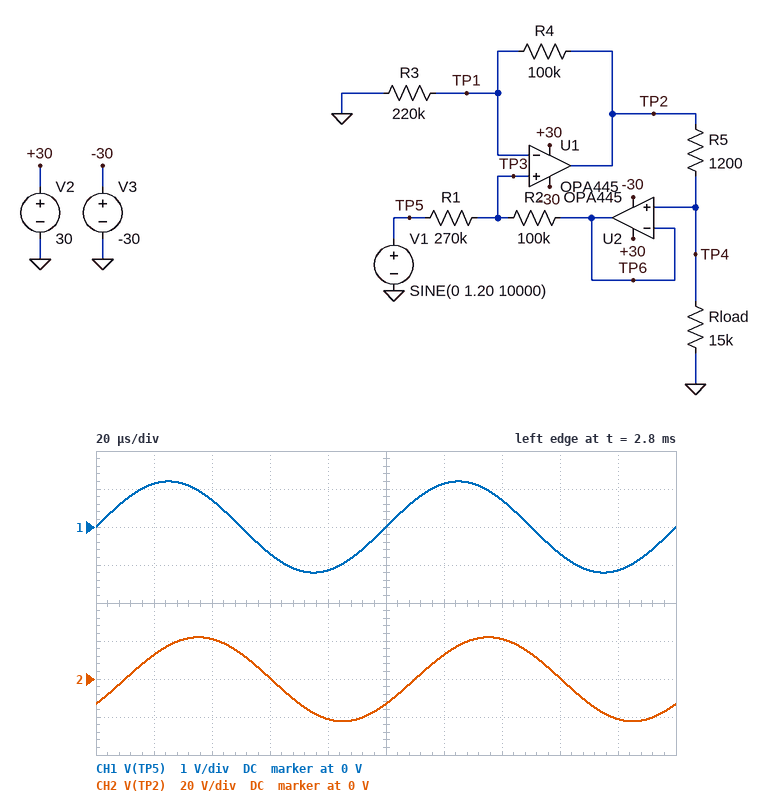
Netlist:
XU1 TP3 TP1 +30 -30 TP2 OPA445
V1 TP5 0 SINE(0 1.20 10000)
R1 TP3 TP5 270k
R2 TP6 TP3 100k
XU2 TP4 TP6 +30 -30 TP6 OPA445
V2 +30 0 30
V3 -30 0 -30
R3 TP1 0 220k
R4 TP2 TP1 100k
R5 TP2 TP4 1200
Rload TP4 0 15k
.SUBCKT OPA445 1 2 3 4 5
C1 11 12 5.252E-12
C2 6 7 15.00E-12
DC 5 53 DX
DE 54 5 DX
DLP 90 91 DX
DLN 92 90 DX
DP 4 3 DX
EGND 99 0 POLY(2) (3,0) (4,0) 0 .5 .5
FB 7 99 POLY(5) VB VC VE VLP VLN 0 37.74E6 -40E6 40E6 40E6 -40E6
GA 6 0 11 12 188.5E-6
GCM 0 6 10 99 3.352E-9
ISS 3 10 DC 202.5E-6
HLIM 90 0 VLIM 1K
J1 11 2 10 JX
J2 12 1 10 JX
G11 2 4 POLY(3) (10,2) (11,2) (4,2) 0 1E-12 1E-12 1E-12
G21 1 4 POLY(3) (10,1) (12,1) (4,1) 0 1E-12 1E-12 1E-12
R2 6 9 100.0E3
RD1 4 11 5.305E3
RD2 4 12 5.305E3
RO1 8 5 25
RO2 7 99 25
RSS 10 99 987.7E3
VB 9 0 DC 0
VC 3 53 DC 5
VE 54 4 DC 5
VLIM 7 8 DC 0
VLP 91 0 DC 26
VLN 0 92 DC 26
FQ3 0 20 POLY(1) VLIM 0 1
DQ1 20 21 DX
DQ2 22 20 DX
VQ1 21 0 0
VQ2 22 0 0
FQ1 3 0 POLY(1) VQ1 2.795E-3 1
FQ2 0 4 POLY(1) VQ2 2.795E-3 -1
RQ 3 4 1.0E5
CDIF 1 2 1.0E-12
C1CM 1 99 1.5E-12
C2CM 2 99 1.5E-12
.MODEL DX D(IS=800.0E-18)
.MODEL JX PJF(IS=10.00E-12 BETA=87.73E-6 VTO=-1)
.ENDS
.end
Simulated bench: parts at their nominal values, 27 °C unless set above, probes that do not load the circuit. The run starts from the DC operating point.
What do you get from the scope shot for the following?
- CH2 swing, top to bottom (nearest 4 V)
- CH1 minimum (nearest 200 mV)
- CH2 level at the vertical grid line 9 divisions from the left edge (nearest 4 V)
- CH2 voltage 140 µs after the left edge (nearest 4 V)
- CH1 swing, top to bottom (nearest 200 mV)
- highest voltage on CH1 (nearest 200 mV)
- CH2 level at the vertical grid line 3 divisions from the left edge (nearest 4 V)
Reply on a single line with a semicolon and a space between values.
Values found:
44 V; -1.2 V; -20 V; 20 V; 2.4 V; 1.2 V; 0 V
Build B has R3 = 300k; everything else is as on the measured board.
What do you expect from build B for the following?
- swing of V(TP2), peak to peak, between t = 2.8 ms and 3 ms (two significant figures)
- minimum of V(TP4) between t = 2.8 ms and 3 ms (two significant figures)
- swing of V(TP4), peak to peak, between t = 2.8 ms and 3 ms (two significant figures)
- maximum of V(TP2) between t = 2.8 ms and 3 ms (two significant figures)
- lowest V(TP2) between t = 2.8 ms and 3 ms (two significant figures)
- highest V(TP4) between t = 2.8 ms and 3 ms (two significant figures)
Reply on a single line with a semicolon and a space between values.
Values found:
8.7 V; -4.0 V; 8.0 V; 4.3 V; -4.3 V; 4.0 V
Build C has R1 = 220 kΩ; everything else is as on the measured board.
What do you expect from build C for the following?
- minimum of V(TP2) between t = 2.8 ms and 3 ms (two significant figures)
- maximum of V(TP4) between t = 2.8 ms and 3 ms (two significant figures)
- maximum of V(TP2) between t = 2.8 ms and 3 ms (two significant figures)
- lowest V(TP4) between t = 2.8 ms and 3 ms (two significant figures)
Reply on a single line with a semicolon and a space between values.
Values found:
-7.3 V; 6.7 V; 7.3 V; -6.7 V
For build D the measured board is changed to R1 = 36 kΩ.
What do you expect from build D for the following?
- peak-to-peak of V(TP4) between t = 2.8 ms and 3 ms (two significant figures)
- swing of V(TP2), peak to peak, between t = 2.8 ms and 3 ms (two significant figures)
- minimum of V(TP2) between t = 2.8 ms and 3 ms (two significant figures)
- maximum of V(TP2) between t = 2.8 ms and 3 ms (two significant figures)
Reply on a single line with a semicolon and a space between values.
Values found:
3.7 V; 4.0 V; -2.0 V; 2.0 V
